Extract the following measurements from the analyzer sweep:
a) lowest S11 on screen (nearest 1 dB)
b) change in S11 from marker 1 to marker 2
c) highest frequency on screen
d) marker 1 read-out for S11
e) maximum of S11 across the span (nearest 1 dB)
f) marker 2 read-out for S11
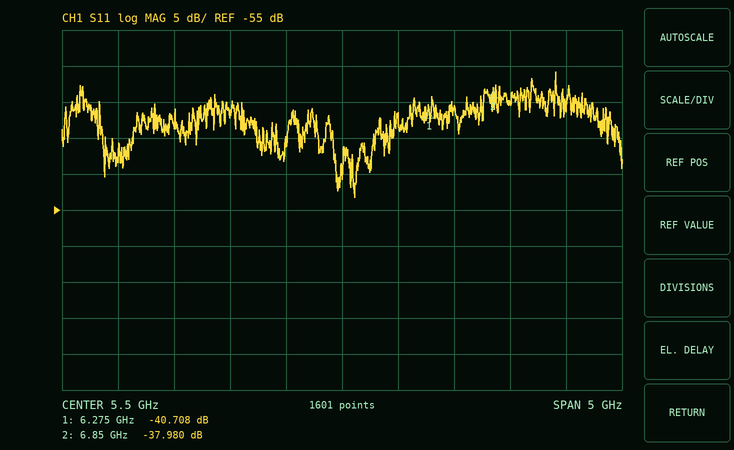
-53 dB
2.728 dB
8 GHz
-40.708 dB
-36 dB
-37.980 dB
